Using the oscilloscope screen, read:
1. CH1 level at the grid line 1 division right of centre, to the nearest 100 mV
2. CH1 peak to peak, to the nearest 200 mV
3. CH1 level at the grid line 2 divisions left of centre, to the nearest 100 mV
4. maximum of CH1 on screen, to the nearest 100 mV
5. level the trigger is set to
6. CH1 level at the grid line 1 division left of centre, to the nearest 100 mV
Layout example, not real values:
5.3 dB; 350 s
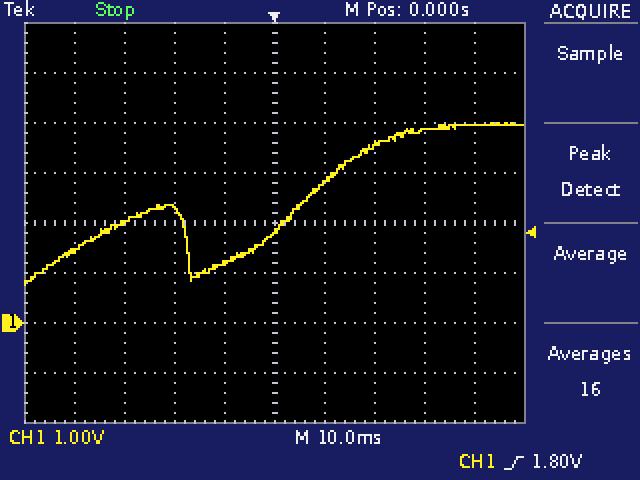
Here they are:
2.8 V; 3.2 V; 2.3 V; 4.0 V; 1.80 V; 1.2 V
